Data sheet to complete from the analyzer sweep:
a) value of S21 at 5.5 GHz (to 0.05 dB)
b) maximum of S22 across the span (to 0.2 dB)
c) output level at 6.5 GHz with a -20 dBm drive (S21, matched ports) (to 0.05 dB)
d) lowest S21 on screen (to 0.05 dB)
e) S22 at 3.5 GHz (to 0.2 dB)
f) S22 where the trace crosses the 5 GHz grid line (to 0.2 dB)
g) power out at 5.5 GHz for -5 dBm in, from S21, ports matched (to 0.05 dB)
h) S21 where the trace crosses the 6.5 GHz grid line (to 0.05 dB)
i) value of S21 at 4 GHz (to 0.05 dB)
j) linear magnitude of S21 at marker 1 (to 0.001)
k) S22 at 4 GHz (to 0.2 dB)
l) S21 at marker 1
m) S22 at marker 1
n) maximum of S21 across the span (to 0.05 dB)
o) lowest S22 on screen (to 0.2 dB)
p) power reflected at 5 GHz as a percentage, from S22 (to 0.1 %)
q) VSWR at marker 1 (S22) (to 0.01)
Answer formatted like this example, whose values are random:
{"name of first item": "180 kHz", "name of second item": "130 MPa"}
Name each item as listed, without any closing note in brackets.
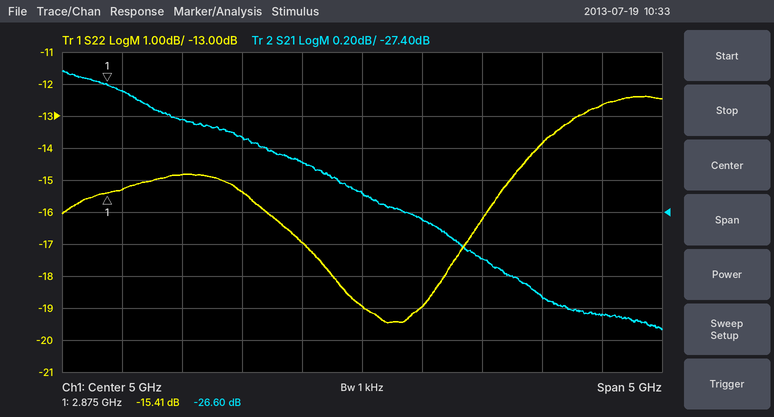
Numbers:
{"value of S21 at 5.5 GHz": "-27.45 dB", "maximum of S22 across the span": "-12.4 dB", "output level at 6.5 GHz with a -20 dBm drive (S21, matched ports)": "-47.95 dBm", "lowest S21 on screen": "-28.15 dB", "S22 at 3.5 GHz": "-14.8 dB", "S22 where the trace crosses the 5 GHz grid line": "-19.0 dB", "power out at 5.5 GHz for -5 dBm in, from S21, ports matched": "-32.45 dBm", "S21 where the trace crosses the 6.5 GHz grid line": "-27.95 dB", "value of S21 at 4 GHz": "-26.95 dB", "linear magnitude of S21 at marker 1": "0.047", "S22 at 4 GHz": "-15.4 dB", "S21 at marker 1": "-26.60 dB", "S22 at marker 1": "-15.41 dB", "maximum of S21 across the span": "-26.50 dB", "lowest S22 on screen": "-19.4 dB", "power reflected at 5 GHz as a percentage, from S22": "1.3 %", "VSWR at marker 1 (S22)": "1.41"}
